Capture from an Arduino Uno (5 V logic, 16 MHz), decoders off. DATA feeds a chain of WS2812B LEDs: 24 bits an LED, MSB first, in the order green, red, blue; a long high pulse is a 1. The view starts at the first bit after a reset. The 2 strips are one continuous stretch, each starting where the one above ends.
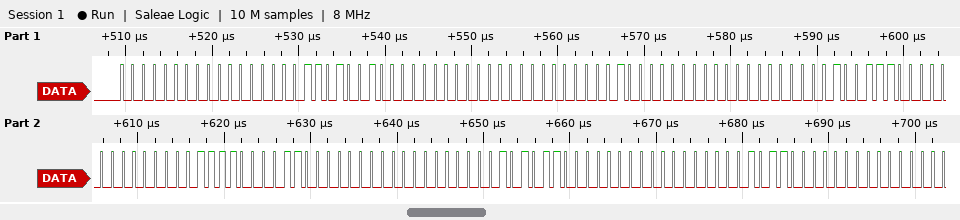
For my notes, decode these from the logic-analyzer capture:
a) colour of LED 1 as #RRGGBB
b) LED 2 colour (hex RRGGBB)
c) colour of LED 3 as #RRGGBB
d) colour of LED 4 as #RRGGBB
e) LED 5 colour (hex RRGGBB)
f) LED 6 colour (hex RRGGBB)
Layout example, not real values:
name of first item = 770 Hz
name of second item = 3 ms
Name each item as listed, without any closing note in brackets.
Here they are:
colour of LED 1 as #RRGGBB = #000069
LED 2 colour = #000002
colour of LED 3 as #RRGGBB = #000027
colour of LED 4 as #RRGGBB = #0300C3
LED 5 colour = #00002B
LED 6 colour = #000058
